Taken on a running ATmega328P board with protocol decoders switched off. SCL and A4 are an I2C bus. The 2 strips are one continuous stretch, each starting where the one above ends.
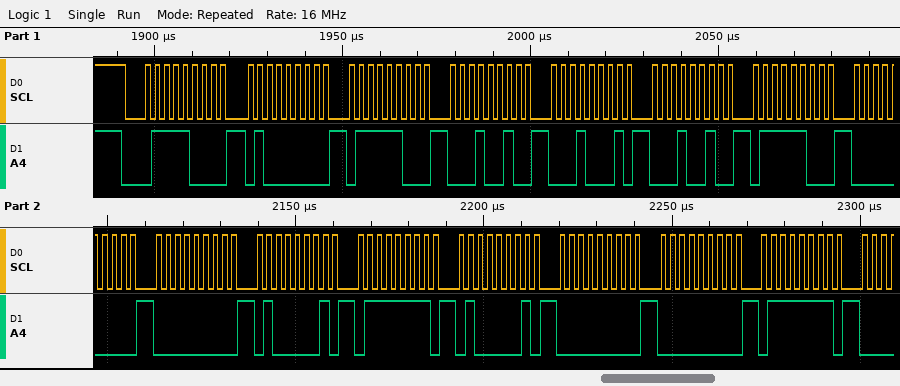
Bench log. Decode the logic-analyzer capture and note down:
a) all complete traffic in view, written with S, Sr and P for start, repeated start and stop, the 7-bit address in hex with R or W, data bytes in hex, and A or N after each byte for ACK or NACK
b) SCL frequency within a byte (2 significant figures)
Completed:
S 3CW A 40 A 7C A 12 A 11 A 12 A 7C A 00 A 00 A 41 A 7F A 41 A 00 A 00 A 7F A
400 kHz
